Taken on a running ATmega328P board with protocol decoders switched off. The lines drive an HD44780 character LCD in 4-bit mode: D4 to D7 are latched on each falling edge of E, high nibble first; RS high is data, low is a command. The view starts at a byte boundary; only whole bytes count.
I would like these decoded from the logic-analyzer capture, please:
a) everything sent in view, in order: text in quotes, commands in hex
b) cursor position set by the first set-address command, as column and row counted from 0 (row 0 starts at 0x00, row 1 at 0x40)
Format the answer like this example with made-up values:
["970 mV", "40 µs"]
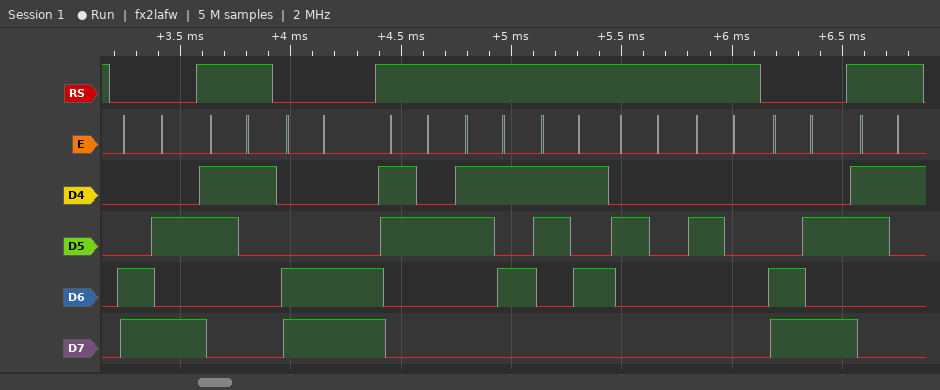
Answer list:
["0xCA \"1\" 0xCC \"255  \" 0xCA \"1\"", "column 10, row 1"]
